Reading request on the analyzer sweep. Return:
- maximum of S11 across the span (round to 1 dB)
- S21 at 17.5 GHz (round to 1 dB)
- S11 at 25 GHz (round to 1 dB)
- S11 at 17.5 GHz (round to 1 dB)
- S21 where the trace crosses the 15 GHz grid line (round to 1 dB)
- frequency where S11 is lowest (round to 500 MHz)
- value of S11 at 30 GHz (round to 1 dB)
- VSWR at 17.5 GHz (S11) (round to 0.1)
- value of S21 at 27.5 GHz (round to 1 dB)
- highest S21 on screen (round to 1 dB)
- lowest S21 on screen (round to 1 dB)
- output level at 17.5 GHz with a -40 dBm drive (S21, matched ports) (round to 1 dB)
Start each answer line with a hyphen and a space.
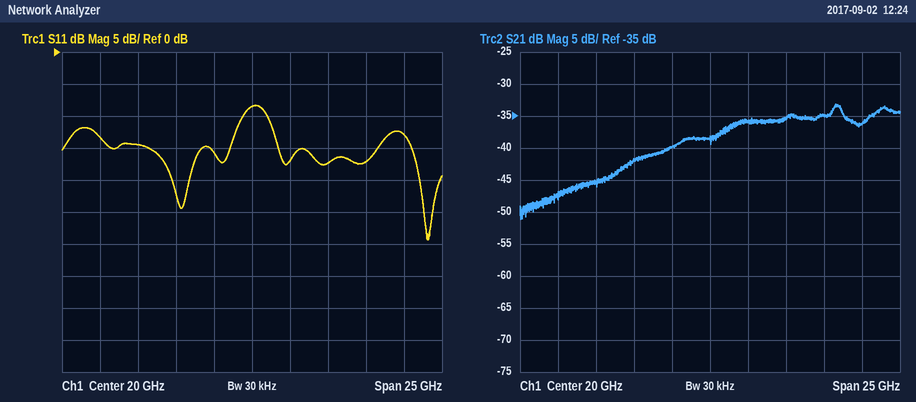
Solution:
- -8 dB
- -40 dB
- -17 dB
- -16 dB
- -42 dB
- 31.5 GHz
- -13 dB
- 1.4
- -35 dB
- -33 dB
- -51 dB
- -80 dBm
